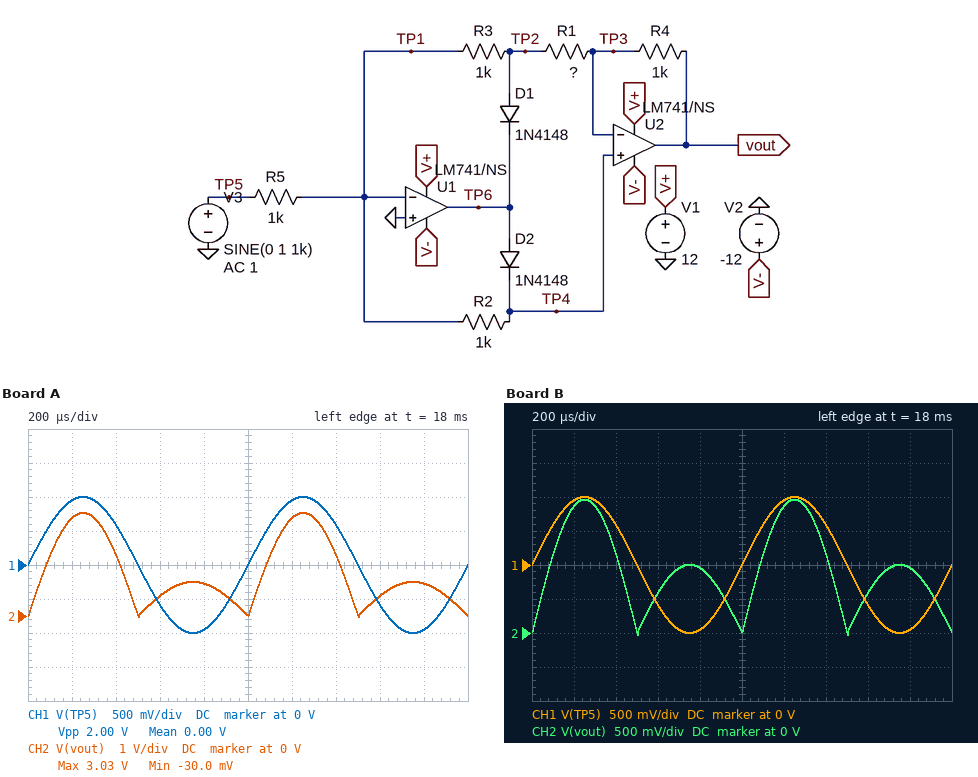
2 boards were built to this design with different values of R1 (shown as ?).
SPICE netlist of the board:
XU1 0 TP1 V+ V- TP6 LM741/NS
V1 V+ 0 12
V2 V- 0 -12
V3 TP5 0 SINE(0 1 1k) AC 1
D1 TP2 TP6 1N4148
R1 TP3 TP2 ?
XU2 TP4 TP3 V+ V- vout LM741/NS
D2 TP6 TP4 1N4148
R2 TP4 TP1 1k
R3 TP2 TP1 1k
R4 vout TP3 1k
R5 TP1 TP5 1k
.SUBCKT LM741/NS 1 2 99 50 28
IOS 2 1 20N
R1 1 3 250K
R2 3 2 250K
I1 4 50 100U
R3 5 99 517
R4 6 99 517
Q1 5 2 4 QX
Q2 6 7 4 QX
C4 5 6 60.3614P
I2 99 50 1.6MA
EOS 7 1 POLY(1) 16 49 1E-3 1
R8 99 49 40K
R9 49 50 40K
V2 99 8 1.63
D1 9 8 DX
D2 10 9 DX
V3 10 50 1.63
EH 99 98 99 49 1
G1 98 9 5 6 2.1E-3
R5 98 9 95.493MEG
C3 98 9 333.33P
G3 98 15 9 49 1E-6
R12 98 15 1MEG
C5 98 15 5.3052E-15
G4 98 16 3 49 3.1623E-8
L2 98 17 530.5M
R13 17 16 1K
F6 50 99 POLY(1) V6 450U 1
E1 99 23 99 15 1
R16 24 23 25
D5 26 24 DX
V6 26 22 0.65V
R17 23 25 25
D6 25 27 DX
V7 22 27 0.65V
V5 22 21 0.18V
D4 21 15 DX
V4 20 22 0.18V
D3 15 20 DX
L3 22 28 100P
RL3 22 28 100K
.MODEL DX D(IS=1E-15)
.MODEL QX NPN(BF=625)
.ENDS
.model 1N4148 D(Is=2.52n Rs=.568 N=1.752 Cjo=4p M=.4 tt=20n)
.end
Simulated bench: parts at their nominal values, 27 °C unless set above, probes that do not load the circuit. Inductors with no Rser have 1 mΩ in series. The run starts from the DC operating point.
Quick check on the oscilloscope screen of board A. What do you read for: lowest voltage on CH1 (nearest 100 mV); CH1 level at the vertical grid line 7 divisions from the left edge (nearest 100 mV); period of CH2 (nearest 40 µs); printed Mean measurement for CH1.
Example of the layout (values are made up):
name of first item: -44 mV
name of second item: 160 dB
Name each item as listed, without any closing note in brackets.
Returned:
lowest voltage on CH1: -1.0 V
CH1 level at the vertical grid line 7 divisions from the left edge: 600 mV
period of CH2: 1.00 ms
printed Mean measurement for CH1: 0.00 V
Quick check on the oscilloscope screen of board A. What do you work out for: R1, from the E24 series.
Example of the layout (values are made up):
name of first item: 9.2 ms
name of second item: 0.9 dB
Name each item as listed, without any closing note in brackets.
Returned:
R1, from the E24 series: 330 Ω
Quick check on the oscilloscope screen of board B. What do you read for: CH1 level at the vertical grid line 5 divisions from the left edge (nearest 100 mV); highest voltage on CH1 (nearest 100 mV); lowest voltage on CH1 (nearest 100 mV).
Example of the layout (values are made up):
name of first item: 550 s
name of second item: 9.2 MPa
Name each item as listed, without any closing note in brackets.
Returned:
CH1 level at the vertical grid line 5 divisions from the left edge: 0 V
highest voltage on CH1: 1.0 V
lowest voltage on CH1: -1.0 V
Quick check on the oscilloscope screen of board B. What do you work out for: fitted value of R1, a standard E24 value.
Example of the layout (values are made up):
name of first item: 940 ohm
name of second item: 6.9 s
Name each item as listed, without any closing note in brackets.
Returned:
fitted value of R1, a standard E24 value: 510 Ω
